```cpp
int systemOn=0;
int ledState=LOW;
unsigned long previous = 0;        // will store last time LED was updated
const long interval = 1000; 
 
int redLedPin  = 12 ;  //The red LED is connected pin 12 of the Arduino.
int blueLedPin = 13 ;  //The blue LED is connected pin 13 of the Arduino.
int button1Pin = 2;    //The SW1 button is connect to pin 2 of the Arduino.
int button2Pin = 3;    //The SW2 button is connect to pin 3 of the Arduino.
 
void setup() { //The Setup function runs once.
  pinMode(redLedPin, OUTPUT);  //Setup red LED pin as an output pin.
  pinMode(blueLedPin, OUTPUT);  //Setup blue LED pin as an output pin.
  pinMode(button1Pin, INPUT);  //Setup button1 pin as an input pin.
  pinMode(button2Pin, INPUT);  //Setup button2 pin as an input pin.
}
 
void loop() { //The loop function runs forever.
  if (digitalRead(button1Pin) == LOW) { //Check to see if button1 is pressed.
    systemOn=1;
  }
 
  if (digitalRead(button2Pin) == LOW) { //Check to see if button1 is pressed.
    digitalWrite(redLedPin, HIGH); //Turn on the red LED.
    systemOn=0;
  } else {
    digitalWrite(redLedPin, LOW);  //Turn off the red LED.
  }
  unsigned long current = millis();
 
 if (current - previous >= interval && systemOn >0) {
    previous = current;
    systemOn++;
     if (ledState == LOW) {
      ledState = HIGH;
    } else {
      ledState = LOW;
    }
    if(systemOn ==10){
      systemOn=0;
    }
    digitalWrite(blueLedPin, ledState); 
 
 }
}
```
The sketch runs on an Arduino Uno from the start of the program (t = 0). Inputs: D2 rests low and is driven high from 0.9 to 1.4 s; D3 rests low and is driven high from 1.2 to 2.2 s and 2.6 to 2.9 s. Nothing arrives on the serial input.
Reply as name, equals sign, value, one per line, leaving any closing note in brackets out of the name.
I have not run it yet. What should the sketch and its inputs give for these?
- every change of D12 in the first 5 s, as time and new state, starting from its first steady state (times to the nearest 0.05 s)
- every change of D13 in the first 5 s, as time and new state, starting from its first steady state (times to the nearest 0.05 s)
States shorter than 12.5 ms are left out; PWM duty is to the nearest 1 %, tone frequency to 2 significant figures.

every change of D12 in the first 5 s, as time and new state, starting from its first steady state = 0 s high; 1.2 s low; 2.2 s high; 2.6 s low; 2.9 s high
every change of D13 in the first 5 s, as time and new state, starting from its first steady state = 0 s low; 1.4 s high; 2.6 s low
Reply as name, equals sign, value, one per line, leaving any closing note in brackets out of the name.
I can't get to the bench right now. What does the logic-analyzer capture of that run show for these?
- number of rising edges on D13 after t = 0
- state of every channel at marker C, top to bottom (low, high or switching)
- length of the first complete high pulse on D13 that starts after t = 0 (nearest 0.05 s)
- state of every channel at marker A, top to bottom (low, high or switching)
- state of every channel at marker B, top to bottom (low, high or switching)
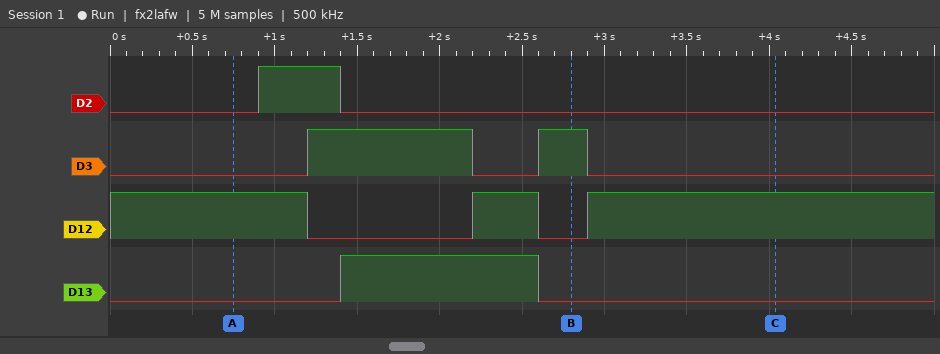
number of rising edges on D13 after t = 0 = 1
state of every channel at marker C, top to bottom = D2 low, D3 low, D12 high, D13 low
length of the first complete high pulse on D13 that starts after t = 0 = 1.20 s
state of every channel at marker A, top to bottom = D2 low, D3 low, D12 high, D13 low
state of every channel at marker B, top to bottom = D2 low, D3 high, D12 low, D13 low
